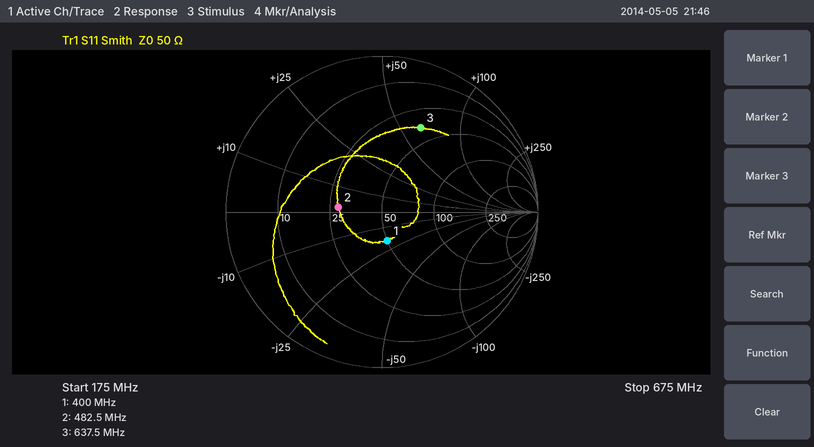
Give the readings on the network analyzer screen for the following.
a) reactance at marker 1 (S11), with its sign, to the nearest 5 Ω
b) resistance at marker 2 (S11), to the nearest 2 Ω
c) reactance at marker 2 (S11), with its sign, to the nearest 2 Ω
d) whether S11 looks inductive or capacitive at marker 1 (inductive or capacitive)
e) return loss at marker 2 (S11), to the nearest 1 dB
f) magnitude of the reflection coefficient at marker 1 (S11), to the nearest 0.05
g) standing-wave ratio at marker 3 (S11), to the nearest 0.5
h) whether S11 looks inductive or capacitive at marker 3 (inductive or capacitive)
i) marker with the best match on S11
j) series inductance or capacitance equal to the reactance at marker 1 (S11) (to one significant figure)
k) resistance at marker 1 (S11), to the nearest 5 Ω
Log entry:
-20 Ω
28 Ω
+2 Ω
capacitive
11 dB
0.20
4.0
inductive
marker 1
20 pF
50 Ω
